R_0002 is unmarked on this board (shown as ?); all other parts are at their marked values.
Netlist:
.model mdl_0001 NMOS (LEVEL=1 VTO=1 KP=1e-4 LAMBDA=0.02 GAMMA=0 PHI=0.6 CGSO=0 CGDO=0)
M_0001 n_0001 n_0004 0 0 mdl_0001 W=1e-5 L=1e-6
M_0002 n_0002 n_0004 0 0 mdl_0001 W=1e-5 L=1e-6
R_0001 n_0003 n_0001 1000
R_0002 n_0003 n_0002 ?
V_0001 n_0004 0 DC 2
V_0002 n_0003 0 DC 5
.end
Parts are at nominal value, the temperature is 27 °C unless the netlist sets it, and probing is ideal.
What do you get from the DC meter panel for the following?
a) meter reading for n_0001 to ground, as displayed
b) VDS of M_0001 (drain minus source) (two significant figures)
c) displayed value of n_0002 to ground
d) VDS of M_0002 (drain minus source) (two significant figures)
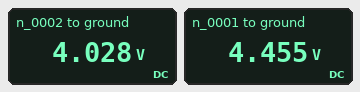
4.455 V
4.5 V
4.028 V
4.0 V
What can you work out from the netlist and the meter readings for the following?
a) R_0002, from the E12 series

1.8 kΩ
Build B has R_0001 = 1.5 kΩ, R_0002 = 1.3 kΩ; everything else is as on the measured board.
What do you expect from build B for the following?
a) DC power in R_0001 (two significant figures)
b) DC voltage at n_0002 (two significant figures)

440 µW
4.3 V
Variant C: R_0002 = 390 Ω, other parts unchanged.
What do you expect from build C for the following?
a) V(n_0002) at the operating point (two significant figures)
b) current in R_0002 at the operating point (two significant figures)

4.8 V
550 µA
